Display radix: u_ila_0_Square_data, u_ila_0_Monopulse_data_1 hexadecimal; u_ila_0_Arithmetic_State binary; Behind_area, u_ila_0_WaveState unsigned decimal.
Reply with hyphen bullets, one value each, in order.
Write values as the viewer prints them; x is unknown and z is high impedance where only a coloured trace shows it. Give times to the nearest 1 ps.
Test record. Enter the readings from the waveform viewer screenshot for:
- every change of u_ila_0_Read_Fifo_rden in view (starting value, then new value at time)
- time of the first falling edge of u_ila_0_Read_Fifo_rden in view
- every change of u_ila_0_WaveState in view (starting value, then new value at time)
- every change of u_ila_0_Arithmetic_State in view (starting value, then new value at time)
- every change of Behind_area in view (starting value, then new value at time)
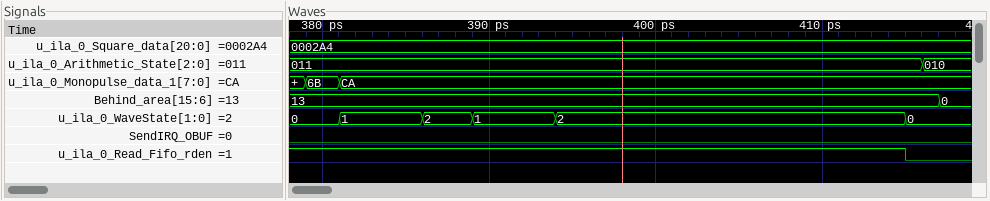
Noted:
- 1, 0 at 415 ps
- 415 ps
- 0, 1 at 381 ps, 2 at 386 ps, 1 at 389 ps, 2 at 394 ps, 0 at 415 ps
- 011, 010 at 416 ps
- 13, 0 at 417 ps
